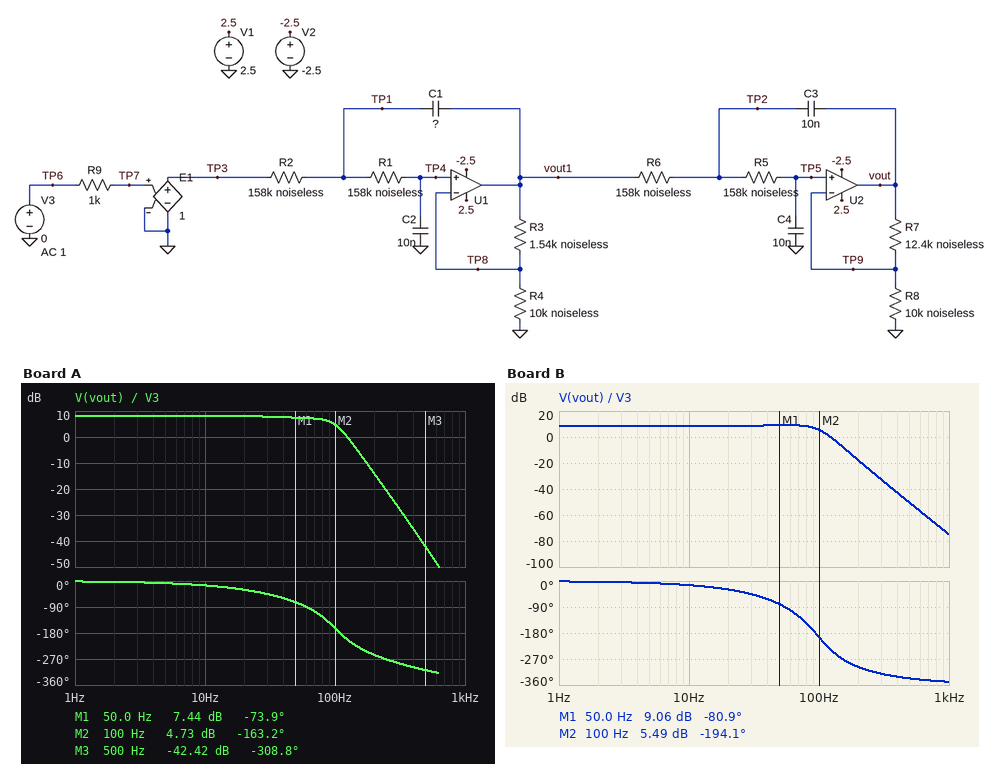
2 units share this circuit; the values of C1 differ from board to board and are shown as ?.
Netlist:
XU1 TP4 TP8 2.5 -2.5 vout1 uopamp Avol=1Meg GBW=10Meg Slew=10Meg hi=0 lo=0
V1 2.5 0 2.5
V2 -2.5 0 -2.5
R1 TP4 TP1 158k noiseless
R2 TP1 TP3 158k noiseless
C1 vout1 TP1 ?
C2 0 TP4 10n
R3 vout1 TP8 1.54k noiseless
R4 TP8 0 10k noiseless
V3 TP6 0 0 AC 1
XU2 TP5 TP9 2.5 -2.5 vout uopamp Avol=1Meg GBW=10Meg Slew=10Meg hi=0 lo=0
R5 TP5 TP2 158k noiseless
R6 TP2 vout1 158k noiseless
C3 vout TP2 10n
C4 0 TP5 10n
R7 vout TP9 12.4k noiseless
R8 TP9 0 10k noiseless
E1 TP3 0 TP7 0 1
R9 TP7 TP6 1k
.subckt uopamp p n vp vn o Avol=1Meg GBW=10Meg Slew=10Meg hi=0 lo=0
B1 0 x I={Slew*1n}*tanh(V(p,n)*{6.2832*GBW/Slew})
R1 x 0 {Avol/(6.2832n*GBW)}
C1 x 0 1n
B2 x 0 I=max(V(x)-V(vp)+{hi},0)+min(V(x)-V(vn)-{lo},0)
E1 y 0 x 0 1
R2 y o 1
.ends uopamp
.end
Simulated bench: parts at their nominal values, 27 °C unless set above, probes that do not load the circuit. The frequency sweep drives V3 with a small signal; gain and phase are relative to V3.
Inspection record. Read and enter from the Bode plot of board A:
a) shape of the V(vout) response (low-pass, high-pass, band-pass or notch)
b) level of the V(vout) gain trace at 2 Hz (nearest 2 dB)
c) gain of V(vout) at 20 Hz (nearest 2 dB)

low-pass
8 dB
8 dB
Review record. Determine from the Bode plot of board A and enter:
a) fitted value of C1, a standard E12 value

4.7 nF
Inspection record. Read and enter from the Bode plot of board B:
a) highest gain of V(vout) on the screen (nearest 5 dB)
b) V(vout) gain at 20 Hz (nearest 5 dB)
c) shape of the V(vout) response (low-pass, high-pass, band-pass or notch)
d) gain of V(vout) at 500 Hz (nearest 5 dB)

10 dB
10 dB
low-pass
-50 dB
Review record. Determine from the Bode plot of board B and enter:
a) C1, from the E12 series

15 nF
